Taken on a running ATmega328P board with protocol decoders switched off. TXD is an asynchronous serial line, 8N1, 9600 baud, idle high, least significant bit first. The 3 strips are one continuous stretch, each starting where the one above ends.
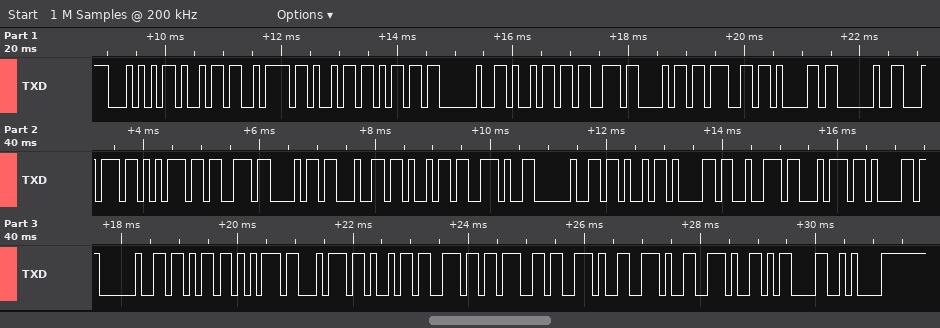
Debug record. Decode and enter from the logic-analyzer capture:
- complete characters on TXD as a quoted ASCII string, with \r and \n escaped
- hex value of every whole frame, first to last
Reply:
"Tizim ishga tushdi. Karta kuting...\r\n"
54 69 7A 69 6D 20 69 73 68 67 61 20 74 75 73 68 64 69 2E 20 4B 61 72 74 61 20 6B 75 74 69 6E 67 2E 2E 2E 0D 0A
